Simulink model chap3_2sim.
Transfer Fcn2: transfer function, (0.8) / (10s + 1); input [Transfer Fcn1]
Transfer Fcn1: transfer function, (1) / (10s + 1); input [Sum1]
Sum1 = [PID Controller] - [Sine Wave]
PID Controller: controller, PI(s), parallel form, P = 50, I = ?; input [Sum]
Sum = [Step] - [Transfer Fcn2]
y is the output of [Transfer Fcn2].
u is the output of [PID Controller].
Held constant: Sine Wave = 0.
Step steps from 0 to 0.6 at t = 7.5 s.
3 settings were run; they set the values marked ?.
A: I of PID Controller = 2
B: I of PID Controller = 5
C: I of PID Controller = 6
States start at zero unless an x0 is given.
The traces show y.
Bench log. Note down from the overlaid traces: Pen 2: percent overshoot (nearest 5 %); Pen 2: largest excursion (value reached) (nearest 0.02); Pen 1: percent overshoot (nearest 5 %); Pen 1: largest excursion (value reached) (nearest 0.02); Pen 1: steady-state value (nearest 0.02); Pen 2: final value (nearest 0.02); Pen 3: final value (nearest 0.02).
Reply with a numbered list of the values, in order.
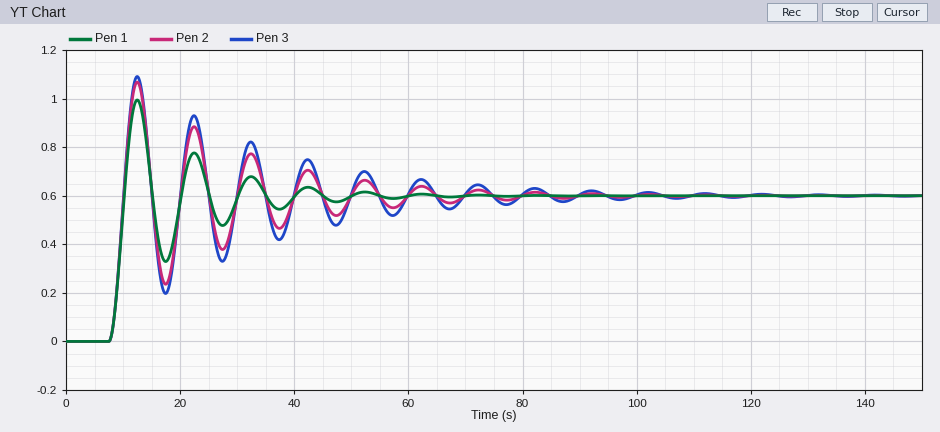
1. 80 %
2. 1.06
3. 65 %
4. 1.00
5. 0.60
6. 0.60
7. 0.60
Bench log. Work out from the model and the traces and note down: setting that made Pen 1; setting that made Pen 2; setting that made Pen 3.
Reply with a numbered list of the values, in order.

1. A
2. B
3. C
